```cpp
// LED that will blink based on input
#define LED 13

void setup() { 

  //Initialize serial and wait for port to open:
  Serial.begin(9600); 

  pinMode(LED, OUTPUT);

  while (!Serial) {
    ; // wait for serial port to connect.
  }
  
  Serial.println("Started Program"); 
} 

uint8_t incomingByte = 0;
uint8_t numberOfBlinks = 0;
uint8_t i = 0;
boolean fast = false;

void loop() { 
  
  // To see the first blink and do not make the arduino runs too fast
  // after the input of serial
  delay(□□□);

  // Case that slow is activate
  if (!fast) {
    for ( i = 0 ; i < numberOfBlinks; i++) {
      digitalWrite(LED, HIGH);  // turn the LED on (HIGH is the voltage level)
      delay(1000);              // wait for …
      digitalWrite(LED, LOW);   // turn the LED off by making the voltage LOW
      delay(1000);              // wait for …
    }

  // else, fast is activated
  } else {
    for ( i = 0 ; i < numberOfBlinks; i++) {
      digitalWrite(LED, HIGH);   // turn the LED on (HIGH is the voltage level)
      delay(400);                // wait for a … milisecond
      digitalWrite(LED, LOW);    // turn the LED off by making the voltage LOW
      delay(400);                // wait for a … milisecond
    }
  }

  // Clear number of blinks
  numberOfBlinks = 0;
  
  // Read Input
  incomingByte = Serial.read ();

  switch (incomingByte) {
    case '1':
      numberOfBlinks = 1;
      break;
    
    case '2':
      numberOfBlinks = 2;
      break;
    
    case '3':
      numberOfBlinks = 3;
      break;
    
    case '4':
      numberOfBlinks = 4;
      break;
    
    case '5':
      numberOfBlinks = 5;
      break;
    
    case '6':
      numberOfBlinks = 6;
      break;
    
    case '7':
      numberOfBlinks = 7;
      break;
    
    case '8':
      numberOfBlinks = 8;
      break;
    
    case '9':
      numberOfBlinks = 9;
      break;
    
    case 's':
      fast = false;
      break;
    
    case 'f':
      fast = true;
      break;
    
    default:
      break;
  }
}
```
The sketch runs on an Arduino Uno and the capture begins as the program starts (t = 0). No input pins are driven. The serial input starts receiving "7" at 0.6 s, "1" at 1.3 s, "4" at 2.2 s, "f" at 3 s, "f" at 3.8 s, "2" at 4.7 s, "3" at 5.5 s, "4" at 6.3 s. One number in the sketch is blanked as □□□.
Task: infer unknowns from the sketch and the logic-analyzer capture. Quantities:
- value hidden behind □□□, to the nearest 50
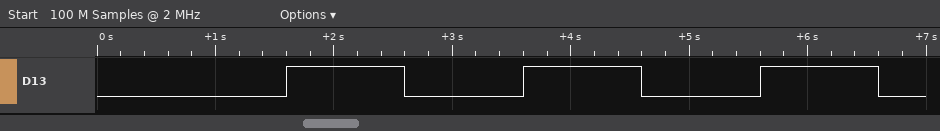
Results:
800
